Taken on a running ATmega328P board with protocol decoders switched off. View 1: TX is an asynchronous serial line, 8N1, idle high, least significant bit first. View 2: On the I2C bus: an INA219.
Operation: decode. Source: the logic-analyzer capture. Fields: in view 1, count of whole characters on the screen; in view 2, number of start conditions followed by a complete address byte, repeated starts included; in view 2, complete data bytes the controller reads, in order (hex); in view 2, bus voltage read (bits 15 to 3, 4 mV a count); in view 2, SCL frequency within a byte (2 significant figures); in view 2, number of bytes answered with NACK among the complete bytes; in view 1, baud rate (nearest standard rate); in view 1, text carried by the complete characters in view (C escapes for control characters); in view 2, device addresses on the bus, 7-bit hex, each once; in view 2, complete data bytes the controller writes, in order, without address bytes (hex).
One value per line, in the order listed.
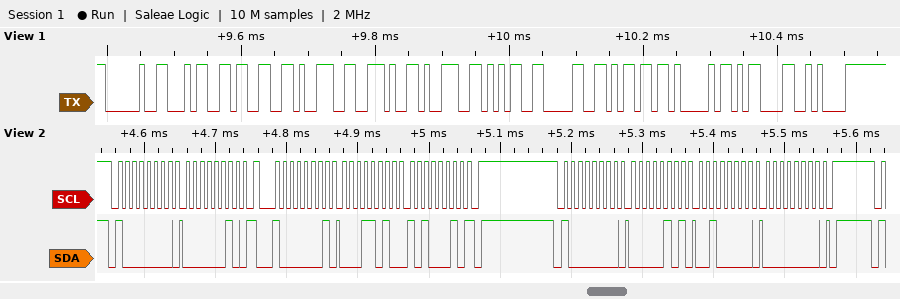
12
3
1A A2
3.408 V
100 kHz
1
115200 baud
" 439.950mA\r\n"
0x40
02 05 20 00
